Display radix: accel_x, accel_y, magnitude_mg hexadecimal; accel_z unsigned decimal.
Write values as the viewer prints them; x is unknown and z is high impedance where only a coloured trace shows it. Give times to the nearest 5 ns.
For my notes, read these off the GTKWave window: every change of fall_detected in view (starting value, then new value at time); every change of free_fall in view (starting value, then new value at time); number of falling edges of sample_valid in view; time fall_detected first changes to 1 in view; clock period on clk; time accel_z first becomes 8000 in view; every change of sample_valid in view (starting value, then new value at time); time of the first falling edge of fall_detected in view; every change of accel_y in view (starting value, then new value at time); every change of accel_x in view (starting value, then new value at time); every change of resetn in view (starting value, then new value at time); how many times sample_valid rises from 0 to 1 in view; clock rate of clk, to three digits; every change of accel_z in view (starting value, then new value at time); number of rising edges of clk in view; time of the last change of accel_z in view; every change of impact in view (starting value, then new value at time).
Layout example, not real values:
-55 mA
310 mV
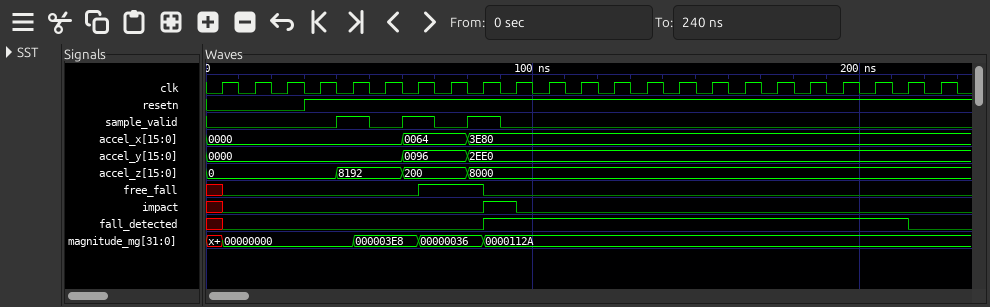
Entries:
x, 0 at 5 ns, 1 at 85 ns, 0 at 215 ns
x, 0 at 5 ns, 1 at 65 ns, 0 at 85 ns
3
85 ns
10 ns
80 ns
0, 1 at 40 ns, 0 at 50 ns, 1 at 60 ns, 0 at 70 ns, 1 at 80 ns, 0 at 90 ns
215 ns
0000, 0096 at 60 ns, 2EE0 at 80 ns
0000, 0064 at 60 ns, 3E80 at 80 ns
0, 1 at 30 ns
3
100 MHz
0, 8192 at 40 ns, 200 at 60 ns, 8000 at 80 ns
23
80 ns
x, 0 at 5 ns, 1 at 85 ns, 0 at 95 ns
